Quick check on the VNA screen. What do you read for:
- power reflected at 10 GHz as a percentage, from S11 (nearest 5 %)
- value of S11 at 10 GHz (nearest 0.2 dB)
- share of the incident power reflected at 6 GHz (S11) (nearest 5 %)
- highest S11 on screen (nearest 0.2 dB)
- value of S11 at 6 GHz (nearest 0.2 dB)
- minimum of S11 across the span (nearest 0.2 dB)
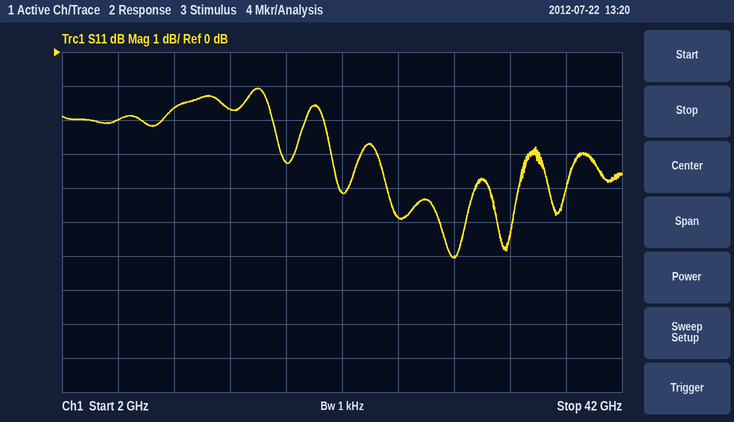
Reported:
70 %
-1.6 dB
65 %
-1.0 dB
-2.0 dB
-6.0 dB
